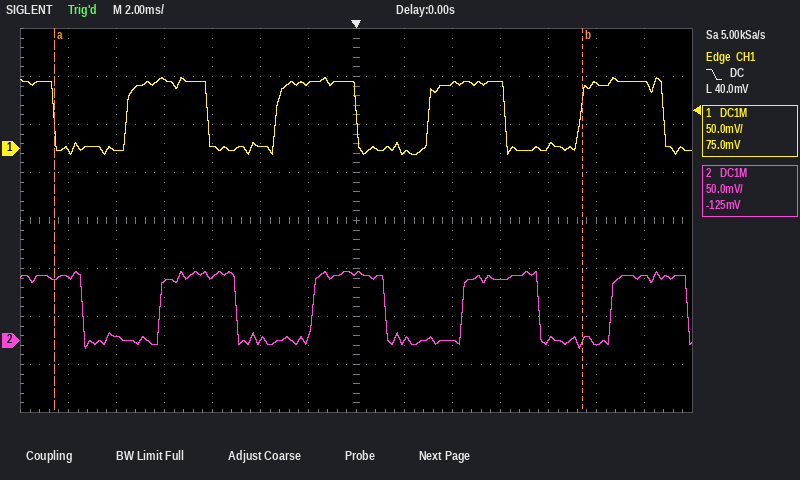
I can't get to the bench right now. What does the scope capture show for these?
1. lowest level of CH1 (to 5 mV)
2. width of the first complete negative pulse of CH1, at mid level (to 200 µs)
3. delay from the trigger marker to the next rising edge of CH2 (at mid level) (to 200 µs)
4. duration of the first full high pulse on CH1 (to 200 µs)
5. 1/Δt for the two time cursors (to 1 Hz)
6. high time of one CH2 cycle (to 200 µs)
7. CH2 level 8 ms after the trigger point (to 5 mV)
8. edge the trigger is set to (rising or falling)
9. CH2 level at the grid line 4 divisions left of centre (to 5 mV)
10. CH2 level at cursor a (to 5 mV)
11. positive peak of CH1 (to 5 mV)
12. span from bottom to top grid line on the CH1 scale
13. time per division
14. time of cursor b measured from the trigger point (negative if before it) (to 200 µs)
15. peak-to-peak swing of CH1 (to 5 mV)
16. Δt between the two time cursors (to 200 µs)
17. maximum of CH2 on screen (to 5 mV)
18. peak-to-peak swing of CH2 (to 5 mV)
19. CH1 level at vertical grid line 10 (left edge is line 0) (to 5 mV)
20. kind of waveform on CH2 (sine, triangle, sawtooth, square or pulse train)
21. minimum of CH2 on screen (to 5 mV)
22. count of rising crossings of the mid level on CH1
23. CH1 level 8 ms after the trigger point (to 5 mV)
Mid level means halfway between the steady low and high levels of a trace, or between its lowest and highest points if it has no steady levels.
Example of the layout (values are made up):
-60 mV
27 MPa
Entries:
-5 mV
3.0 ms
4.4 ms
3.4 ms
45 Hz
3.2 ms
0 mV
falling
60 mV
65 mV
75 mV
400 mV
2 ms
+9.4 ms
80 mV
22.0 ms
70 mV
80 mV
70 mV
square
-10 mV
4
0 mV
